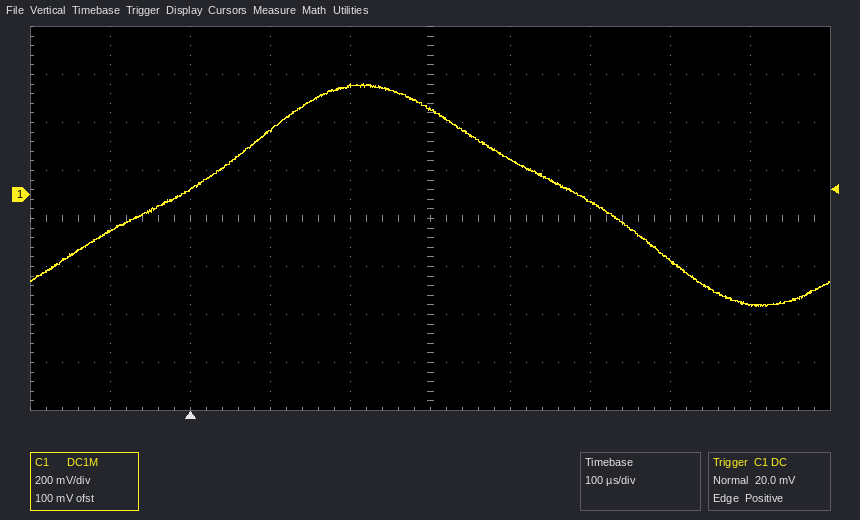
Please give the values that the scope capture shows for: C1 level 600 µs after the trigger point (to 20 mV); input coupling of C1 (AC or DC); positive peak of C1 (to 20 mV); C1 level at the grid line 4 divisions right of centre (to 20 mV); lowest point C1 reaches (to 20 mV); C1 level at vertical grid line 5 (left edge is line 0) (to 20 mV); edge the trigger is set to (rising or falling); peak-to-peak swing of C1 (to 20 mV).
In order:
-280 mV
DC
460 mV
-460 mV
-460 mV
360 mV
rising
920 mV
